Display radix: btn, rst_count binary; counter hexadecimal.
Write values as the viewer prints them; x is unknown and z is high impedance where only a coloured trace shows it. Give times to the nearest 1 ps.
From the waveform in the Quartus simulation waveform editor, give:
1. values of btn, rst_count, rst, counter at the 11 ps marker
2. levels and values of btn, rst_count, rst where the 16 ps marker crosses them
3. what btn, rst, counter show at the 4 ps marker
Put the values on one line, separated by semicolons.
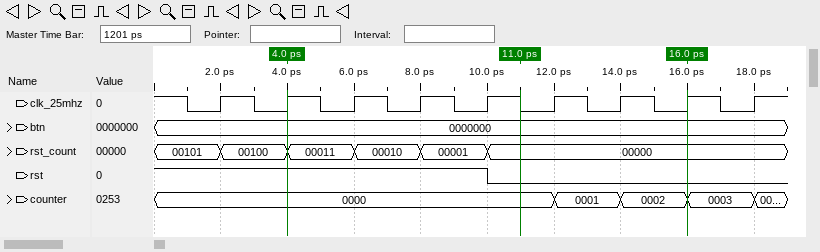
btn=0000000, rst_count=00000, rst=0, counter=0000; btn=0000000, rst_count=00000, rst=0; btn=0000000, rst=1, counter=0000
